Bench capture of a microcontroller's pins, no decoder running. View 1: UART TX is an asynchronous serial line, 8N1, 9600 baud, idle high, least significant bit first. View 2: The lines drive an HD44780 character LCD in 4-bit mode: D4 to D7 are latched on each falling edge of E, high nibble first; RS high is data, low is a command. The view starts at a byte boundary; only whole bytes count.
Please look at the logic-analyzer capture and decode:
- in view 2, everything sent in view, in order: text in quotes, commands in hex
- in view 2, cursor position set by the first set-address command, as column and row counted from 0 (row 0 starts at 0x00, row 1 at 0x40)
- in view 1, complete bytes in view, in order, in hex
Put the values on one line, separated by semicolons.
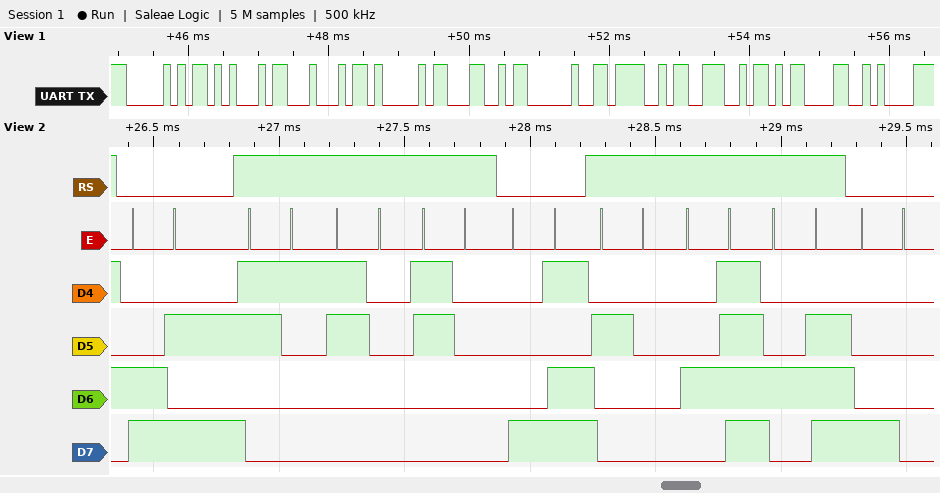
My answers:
0xCA "100" 0x8D " ON" 0x80; column 10, row 1; 50 45 44 41 4C 20 4F 4E 0D 0A
